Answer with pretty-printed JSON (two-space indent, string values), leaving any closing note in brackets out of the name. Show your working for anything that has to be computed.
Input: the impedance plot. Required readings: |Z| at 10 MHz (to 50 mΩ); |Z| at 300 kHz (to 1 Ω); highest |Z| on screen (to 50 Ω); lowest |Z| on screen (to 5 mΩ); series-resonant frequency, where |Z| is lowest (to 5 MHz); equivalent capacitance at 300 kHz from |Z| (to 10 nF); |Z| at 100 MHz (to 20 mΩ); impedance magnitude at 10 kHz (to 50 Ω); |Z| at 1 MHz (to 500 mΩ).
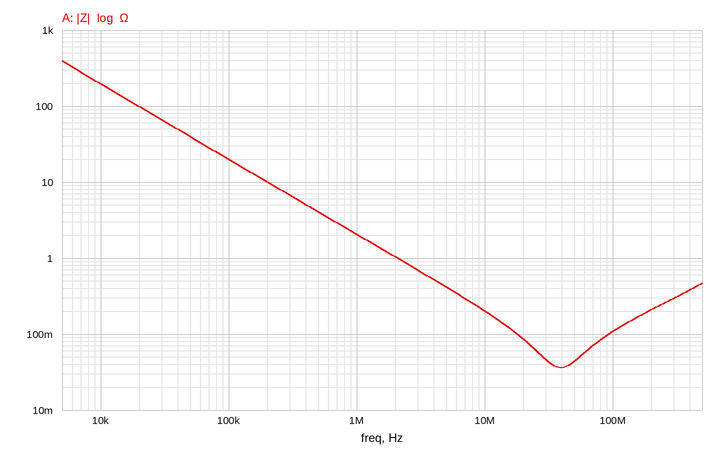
{
  "|Z| at 10 MHz": "200 mΩ",
  "|Z| at 300 kHz": "7 Ω",
  "highest |Z| on screen": "400 Ω",
  "lowest |Z| on screen": "35 mΩ",
  "series-resonant frequency, where |Z| is lowest": "40 MHz",
  "equivalent capacitance at 300 kHz from |Z|": "C = 1/(2π × 300 kHz × 7 Ω) ≈ 75.8 nF, so 80 nF to the nearest 10 nF",
  "|Z| at 100 MHz": "100 mΩ",
  "impedance magnitude at 10 kHz": "200 Ω",
  "|Z| at 1 MHz": "2.0 Ω"
}
